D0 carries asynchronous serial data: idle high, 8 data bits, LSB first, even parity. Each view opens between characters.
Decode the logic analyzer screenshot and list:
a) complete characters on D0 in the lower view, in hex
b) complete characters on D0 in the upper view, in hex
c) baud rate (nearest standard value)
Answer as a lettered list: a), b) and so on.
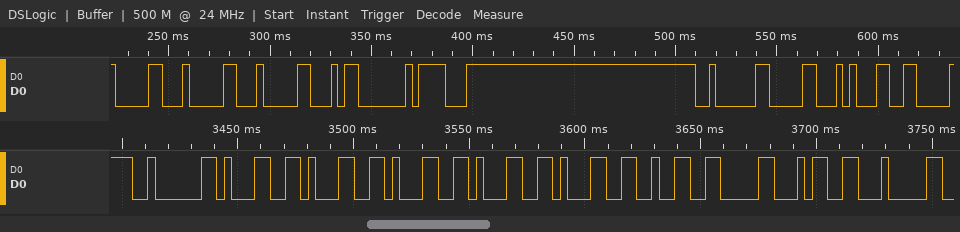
a) 02, 31, 31, 31, 31, 31, 32, 30, 33
b) 30, 30, 30, 03, 8F, 02, 30, 31
c) 300 baud
